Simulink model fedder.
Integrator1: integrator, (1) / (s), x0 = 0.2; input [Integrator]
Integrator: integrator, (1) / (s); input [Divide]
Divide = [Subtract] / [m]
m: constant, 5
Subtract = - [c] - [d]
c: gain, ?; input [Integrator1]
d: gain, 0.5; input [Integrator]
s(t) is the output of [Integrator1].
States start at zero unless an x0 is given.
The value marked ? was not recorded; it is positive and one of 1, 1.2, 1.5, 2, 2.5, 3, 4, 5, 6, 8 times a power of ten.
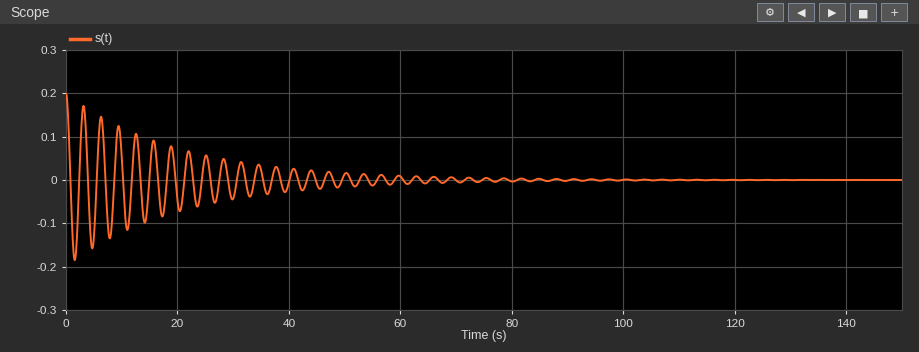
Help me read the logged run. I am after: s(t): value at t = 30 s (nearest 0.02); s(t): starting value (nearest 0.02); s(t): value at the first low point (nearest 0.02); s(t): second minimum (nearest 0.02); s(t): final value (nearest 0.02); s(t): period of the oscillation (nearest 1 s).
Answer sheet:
-0.04
0.20
-0.18
-0.16
0.00
3 s
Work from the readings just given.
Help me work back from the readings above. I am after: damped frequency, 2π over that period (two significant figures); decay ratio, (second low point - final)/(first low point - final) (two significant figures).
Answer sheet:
2.1 rad/s
0.89
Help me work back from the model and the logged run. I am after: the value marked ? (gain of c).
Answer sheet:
20
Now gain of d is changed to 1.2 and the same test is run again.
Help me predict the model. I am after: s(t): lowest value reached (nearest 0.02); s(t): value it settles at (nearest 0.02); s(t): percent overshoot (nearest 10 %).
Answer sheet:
-0.16
0.00
80 %
